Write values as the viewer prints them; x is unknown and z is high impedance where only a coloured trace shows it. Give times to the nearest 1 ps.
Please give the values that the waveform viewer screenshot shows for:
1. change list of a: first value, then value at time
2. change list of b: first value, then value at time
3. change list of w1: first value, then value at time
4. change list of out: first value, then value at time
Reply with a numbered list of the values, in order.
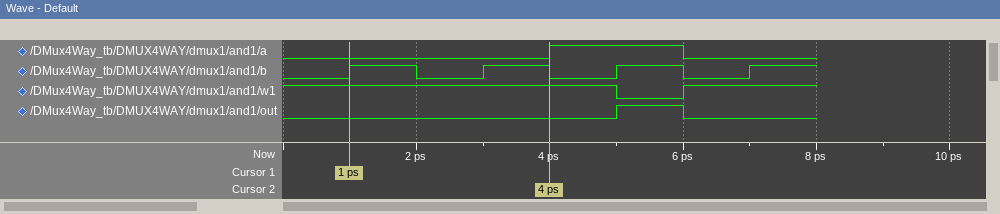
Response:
1. 0, 1 at 4 ps, 0 at 6 ps
2. 0, 1 at 1 ps, 0 at 2 ps, 1 at 3 ps, 0 at 4 ps, 1 at 5 ps, 0 at 6 ps, 1 at 7 ps
3. 1, 0 at 5 ps, 1 at 6 ps
4. 0, 1 at 5 ps, 0 at 6 ps
